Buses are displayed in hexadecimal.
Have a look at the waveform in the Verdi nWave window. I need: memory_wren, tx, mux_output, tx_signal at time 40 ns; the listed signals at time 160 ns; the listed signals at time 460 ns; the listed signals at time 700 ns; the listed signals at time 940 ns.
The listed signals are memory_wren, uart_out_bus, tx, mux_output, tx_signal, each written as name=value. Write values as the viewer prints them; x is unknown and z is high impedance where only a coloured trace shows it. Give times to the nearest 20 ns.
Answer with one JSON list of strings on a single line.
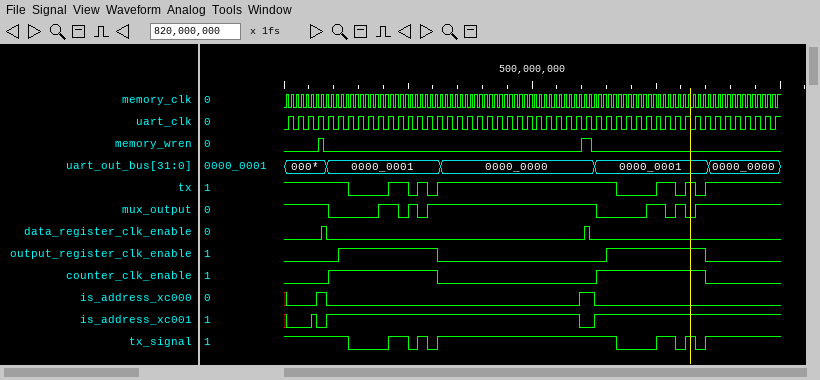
["memory_wren=0, tx=1, mux_output=1, tx_signal=1", "memory_wren=0, uart_out_bus=0000_0001, tx=0, mux_output=0, tx_signal=0", "memory_wren=0, uart_out_bus=0000_0000, tx=1, mux_output=1, tx_signal=1", "memory_wren=0, uart_out_bus=0000_0001, tx=0, mux_output=0, tx_signal=0", "memory_wren=0, uart_out_bus=0000_0000, tx=1, mux_output=1, tx_signal=1"]
